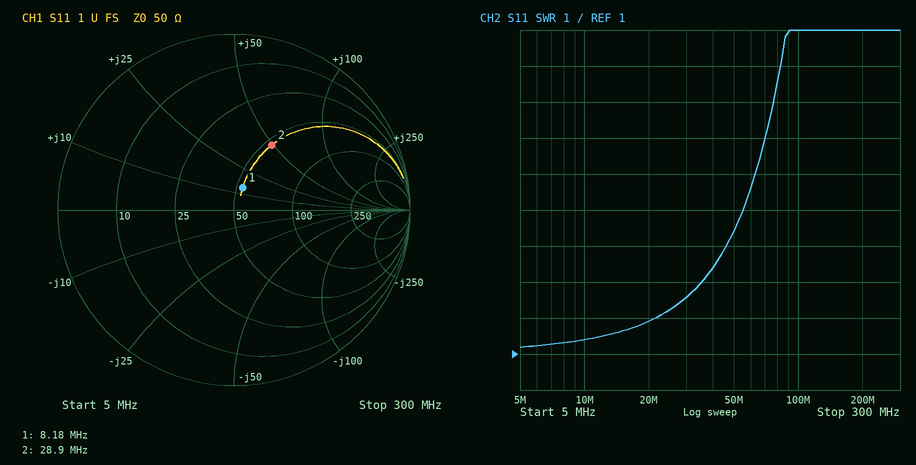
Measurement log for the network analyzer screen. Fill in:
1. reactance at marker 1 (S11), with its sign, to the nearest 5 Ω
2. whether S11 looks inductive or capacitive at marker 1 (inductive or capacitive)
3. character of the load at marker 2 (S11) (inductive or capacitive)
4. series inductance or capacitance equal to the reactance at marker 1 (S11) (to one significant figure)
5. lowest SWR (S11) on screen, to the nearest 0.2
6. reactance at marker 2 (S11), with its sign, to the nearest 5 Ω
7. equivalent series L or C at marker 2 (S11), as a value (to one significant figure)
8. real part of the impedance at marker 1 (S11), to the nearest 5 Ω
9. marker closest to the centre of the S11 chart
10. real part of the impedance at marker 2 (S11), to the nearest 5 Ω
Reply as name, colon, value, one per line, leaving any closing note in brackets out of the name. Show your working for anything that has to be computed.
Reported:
reactance at marker 1 (S11), with its sign, to the nearest 5 Ω: +15 Ω
whether S11 looks inductive or capacitive at marker 1: inductive
character of the load at marker 2 (S11): inductive
series inductance or capacitance equal to the reactance at marker 1 (S11): L = 15 Ω/(2π × 8.18 MHz) ≈ 292 nH, so 300 nH to one significant figure
lowest SWR (S11) on screen, to the nearest 0.2: 1.2
reactance at marker 2 (S11), with its sign, to the nearest 5 Ω: +50 Ω
equivalent series L or C at marker 2 (S11), as a value: L = 50 Ω/(2π × 28.9 MHz) ≈ 275 nH, so 300 nH to one significant figure
real part of the impedance at marker 1 (S11), to the nearest 5 Ω: 55 Ω
marker closest to the centre of the S11 chart: marker 1
real part of the impedance at marker 2 (S11), to the nearest 5 Ω: 55 Ω
